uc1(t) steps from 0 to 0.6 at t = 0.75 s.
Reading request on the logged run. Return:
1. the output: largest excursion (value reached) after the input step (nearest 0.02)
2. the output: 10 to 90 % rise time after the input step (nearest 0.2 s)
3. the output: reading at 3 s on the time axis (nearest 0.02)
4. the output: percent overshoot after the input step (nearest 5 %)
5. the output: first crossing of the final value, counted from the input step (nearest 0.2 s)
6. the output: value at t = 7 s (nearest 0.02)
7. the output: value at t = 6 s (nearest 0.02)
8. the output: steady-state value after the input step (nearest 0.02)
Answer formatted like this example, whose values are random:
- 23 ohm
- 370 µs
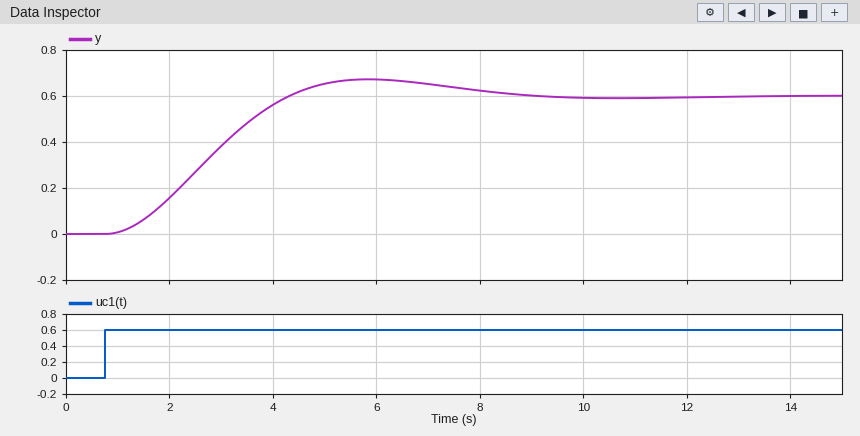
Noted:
- 0.68
- 2.4 s
- 0.38
- 10 %
- 3.6 s
- 0.66
- 0.68
- 0.60
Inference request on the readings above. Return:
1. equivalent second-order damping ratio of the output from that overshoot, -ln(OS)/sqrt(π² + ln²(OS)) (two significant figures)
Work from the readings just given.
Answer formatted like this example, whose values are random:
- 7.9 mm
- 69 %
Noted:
- 0.59
